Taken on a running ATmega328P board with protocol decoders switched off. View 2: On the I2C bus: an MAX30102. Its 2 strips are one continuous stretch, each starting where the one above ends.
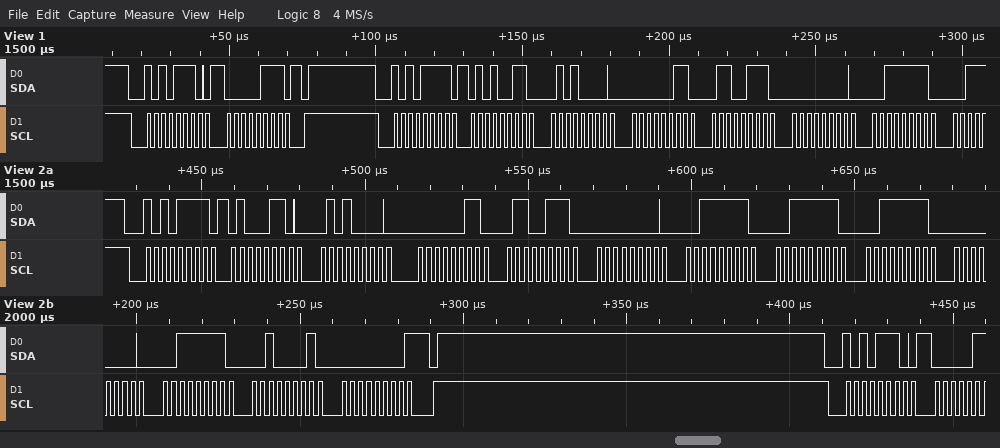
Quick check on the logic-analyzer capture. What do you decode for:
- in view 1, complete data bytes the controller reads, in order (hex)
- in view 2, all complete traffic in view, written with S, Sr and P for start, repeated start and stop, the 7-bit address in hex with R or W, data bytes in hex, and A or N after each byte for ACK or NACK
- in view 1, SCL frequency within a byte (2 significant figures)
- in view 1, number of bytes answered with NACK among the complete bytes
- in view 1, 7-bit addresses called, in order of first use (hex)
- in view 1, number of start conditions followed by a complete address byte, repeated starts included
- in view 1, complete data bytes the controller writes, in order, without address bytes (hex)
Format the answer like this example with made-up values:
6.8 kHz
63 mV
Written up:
53 50 03 67 00 3F
S 57R A 46 A 50 A 03 A 67 A 00 A 3F A 3F A 3F A 00 A 3F A 21 A 00 N P S 57W A
400 kHz
0
0x57
2
07
